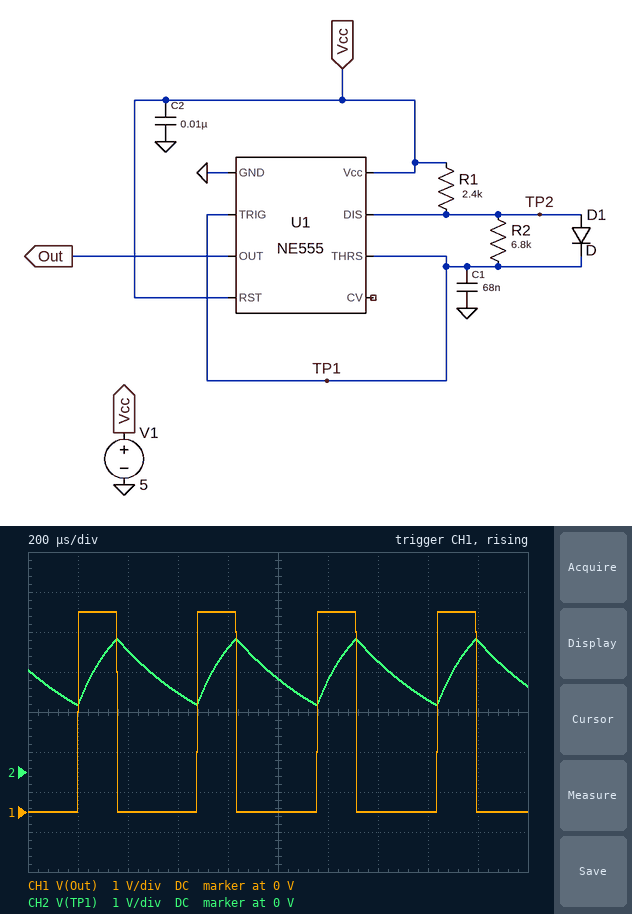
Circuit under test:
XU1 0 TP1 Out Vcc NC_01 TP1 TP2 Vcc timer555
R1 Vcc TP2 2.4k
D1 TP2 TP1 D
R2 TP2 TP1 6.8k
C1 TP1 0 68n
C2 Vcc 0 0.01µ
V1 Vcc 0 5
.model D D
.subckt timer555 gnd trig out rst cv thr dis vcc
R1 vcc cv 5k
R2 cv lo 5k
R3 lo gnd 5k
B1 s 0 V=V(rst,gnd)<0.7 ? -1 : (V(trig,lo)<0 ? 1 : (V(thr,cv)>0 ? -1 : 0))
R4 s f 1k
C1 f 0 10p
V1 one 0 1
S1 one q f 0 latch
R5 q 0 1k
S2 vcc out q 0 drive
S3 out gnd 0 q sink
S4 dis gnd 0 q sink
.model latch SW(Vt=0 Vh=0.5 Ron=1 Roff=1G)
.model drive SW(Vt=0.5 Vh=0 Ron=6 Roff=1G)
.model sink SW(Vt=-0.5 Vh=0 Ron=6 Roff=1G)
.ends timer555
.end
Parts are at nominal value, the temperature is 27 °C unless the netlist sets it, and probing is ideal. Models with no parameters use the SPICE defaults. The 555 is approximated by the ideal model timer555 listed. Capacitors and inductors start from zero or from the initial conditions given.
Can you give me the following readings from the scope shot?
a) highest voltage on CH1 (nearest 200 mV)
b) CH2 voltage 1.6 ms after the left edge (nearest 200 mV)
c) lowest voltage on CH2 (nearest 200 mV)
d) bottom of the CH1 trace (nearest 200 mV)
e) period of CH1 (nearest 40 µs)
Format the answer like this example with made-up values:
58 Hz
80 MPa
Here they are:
5.0 V
1.8 V
1.6 V
0 V
480 µs
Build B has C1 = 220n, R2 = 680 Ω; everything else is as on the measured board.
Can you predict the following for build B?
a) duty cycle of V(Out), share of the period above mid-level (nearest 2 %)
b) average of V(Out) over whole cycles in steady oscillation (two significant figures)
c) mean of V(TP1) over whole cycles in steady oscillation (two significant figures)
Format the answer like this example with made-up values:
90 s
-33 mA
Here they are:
82 %
4.1 V
2.6 V
